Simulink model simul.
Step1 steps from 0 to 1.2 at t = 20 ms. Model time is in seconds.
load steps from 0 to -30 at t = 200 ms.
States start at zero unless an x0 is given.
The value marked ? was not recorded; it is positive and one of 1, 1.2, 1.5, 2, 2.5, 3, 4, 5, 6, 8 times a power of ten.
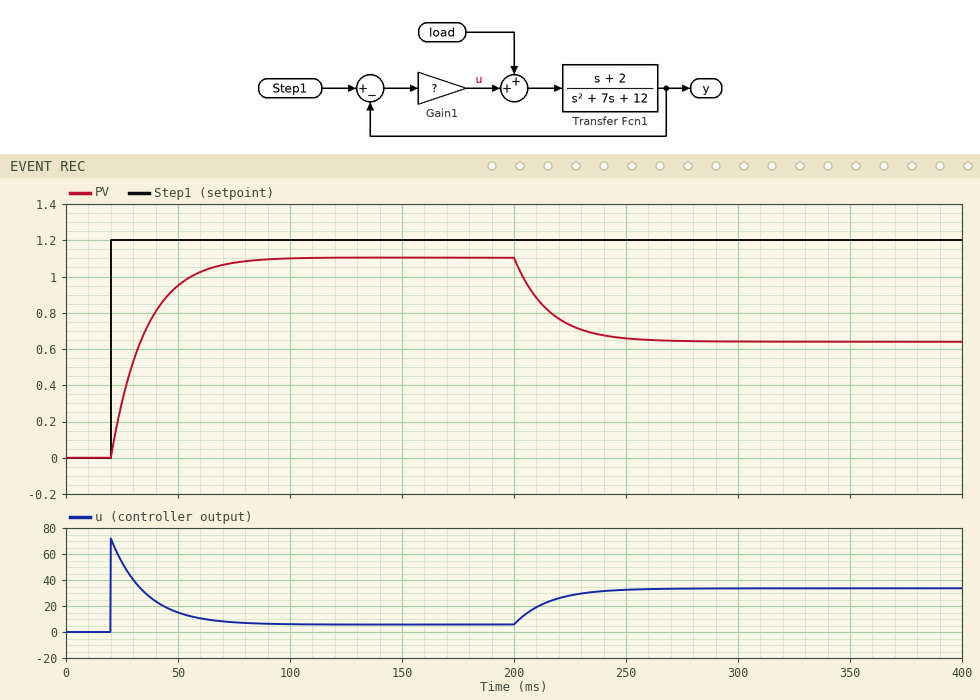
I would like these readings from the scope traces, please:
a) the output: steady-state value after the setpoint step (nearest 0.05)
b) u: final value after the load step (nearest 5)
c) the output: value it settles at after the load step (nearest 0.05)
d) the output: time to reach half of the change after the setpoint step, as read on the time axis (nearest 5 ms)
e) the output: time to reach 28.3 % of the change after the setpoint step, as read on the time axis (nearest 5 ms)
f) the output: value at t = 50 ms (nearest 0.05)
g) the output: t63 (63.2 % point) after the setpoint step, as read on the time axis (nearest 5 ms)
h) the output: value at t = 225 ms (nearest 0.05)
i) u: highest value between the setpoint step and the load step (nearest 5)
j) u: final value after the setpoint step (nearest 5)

1.10
35
0.65
30 ms
25 ms
0.95
35 ms
0.75
70
5
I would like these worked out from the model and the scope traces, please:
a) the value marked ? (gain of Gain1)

60
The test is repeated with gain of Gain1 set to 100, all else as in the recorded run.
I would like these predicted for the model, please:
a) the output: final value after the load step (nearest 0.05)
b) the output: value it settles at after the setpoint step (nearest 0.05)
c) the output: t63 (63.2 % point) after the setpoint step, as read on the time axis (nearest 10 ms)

0.85
1.15
30 ms
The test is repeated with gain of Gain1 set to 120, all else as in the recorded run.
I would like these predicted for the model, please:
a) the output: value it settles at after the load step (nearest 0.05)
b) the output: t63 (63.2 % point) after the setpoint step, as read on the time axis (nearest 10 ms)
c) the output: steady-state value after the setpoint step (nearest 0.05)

0.90
30 ms
1.15
